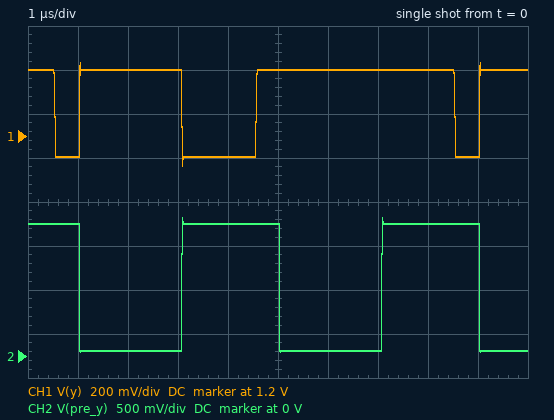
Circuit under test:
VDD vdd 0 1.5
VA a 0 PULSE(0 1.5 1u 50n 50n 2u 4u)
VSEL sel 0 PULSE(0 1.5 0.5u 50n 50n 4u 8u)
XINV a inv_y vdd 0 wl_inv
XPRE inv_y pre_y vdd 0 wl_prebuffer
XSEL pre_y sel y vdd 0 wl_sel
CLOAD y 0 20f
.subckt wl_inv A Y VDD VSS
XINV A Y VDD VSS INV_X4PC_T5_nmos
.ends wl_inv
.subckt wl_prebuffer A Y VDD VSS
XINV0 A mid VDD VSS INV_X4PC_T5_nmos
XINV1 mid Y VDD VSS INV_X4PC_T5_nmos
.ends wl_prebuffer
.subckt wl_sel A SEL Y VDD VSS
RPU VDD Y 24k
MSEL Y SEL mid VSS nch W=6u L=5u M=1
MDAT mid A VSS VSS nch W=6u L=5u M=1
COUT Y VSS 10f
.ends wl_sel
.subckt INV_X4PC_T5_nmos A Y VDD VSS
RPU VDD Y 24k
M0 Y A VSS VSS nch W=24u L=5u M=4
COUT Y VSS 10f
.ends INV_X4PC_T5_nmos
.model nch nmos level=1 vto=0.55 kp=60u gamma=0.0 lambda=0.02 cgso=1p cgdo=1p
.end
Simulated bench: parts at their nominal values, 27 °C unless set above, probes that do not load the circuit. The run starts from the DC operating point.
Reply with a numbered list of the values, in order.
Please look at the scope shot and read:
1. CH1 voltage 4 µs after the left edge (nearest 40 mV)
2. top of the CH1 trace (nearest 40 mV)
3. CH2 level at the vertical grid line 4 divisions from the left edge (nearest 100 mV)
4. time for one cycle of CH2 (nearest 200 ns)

1. 1.12 V
2. 1.52 V
3. 1.5 V
4. 4.0 µs
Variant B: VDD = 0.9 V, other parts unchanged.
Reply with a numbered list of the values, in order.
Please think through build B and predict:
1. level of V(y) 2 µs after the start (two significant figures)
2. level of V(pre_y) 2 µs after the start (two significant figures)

1. 900 mV
2. 96 mV
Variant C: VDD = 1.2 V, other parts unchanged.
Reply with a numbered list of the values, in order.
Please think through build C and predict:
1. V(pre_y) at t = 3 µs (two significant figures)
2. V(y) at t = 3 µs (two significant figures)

1. 66 mV
2. 1.2 V
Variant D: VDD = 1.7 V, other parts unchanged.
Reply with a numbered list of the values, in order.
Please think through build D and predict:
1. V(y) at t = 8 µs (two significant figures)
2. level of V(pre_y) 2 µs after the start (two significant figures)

1. 1.7 V
2. 53 mV
